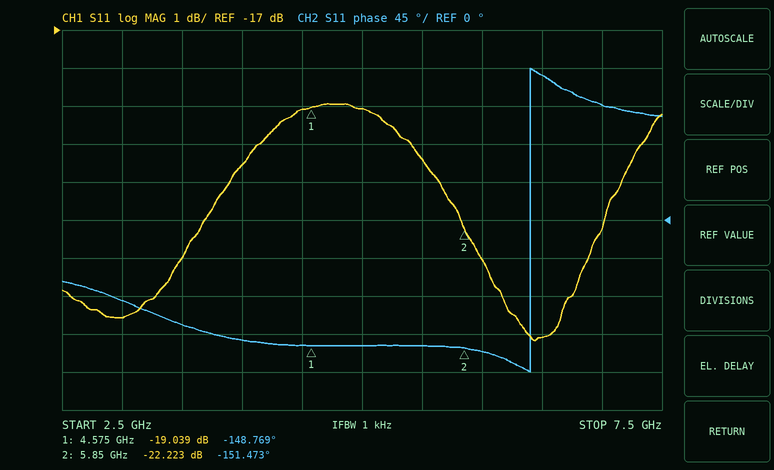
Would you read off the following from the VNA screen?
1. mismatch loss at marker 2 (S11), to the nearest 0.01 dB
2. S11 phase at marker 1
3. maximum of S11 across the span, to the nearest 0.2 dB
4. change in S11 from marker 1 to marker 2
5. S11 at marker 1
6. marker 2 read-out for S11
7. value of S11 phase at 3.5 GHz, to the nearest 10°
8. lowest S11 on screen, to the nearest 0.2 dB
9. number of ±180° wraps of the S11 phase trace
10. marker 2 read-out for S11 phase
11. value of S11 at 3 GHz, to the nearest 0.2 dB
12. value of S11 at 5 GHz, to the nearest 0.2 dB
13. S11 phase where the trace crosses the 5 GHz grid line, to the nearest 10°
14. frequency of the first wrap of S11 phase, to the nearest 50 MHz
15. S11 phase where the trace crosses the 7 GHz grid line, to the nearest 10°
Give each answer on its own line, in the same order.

0.03 dB
-148.769°
-19.0 dB
-3.184 dB
-19.039 dB
-22.223 dB
-120°
-25.2 dB
1
-151.473°
-24.6 dB
-19.0 dB
-150°
6.40 GHz
140°
